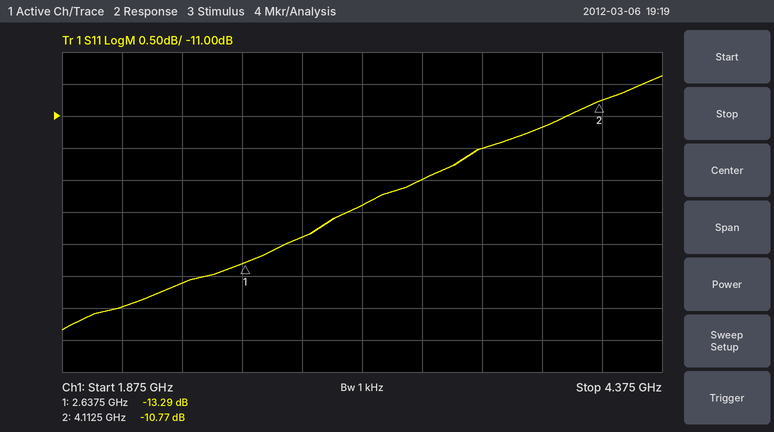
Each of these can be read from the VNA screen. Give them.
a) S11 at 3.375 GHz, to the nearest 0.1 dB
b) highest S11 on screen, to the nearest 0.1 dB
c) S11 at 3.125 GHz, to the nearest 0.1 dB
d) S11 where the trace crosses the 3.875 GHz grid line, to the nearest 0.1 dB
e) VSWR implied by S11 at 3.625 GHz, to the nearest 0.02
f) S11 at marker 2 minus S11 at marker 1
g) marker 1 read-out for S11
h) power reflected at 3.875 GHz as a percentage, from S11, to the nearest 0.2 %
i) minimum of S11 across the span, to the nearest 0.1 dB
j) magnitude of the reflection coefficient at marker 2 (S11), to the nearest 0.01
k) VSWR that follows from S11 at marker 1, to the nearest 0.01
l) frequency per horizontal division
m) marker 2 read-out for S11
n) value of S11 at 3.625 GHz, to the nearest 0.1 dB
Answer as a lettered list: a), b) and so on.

a) -12.0 dB
b) -10.4 dB
c) -12.4 dB
d) -11.2 dB
e) 1.72
f) 2.52 dB
g) -13.29 dB
h) 7.6 %
i) -14.3 dB
j) 0.29
k) 1.55
l) 250 MHz
m) -10.77 dB
n) -11.5 dB
